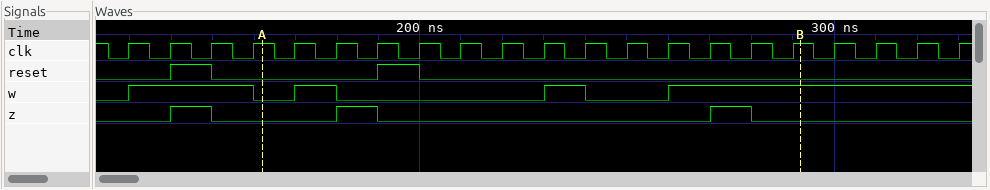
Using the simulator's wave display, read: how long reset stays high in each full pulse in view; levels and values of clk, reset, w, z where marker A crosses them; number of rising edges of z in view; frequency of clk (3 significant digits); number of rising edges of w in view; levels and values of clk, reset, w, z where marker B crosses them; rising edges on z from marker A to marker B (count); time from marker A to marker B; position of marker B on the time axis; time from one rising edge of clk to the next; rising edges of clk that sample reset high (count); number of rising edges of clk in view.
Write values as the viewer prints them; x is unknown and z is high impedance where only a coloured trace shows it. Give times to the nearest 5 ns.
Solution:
10 ns, 10 ns
clk=1, reset=0, w=0, z=0
3
100 MHz
4
clk=1, reset=0, w=1, z=0
2
130 ns
290 ns
10 ns
2
21
